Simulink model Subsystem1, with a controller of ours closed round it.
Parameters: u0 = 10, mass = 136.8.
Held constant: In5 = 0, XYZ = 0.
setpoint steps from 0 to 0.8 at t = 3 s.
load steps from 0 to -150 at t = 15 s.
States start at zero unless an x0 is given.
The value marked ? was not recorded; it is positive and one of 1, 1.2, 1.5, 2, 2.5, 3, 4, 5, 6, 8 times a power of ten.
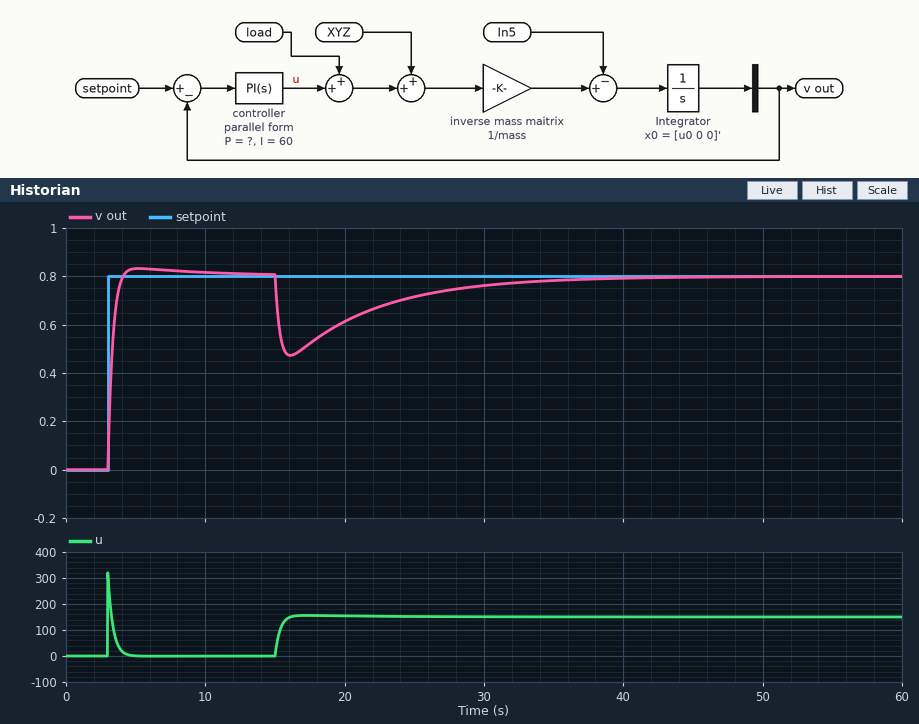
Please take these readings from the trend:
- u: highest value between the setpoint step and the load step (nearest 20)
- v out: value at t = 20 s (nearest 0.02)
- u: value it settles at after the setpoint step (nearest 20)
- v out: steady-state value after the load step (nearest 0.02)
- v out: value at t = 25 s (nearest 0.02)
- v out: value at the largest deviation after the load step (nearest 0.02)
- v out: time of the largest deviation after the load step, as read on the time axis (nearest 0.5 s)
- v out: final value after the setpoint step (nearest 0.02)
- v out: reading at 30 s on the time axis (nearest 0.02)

320
0.62
0
0.80
0.72
0.48
16.0 s
0.80
0.76
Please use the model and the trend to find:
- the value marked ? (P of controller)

400
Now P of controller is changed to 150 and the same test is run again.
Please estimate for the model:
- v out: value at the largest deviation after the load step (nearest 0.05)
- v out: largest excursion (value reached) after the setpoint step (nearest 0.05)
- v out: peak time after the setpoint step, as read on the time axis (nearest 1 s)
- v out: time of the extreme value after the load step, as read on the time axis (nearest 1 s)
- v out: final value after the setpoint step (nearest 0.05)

0.10
0.95
6 s
17 s
0.80
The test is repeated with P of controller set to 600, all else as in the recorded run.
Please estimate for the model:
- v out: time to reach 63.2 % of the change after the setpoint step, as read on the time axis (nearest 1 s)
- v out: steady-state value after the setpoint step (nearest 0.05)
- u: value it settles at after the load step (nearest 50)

3 s
0.80
150
